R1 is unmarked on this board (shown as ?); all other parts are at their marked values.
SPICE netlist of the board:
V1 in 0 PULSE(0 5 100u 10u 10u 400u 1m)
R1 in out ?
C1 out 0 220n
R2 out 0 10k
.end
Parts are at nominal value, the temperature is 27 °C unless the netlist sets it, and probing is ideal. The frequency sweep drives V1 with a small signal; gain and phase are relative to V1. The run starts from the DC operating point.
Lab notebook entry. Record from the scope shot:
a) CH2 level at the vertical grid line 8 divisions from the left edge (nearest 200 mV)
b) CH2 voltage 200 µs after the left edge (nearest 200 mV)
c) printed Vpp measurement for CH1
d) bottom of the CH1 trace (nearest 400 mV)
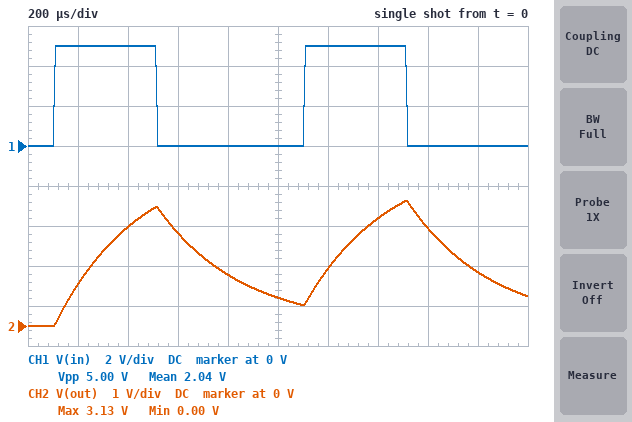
2.4 V
1.0 V
5.00 V
0 V
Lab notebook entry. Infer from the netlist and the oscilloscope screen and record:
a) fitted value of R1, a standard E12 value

1.8 kΩ
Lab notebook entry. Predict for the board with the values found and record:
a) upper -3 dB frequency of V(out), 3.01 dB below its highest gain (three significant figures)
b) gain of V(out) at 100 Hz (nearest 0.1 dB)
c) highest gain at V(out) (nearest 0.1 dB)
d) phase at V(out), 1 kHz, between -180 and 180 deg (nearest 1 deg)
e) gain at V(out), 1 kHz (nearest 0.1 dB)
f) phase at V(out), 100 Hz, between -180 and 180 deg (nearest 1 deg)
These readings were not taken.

474 Hz
-1.6 dB
-1.4 dB
-65 deg
-8.8 dB
-12 deg
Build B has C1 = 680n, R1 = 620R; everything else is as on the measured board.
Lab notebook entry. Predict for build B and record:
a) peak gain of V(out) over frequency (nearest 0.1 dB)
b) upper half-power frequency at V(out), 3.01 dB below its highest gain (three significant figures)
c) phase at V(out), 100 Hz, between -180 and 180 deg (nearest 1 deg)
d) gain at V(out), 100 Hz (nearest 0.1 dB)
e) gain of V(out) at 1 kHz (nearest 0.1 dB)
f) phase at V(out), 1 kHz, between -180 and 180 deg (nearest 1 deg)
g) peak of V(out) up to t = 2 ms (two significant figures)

-0.5 dB
401 Hz
-14 deg
-0.8 dB
-9.1 dB
-68 deg
3.3 V
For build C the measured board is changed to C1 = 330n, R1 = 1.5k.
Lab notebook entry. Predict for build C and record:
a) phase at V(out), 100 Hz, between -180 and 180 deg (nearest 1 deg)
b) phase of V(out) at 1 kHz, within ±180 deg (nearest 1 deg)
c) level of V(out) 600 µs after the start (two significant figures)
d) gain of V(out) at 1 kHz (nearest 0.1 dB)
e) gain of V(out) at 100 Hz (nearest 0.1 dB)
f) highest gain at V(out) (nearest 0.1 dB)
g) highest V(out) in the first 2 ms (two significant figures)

-15 deg
-70 deg
2.2 V
-10.4 dB
-1.5 dB
-1.2 dB
2.9 V
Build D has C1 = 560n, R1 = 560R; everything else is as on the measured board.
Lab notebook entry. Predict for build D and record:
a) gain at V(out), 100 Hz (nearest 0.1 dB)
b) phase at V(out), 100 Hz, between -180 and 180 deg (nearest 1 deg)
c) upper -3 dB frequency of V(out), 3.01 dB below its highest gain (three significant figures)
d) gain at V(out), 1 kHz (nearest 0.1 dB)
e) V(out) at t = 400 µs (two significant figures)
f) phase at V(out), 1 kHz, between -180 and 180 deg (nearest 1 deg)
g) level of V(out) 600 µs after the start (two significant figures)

-0.6 dB
-11 deg
536 Hz
-7.0 dB
3.0 V
-62 deg
2.7 V
